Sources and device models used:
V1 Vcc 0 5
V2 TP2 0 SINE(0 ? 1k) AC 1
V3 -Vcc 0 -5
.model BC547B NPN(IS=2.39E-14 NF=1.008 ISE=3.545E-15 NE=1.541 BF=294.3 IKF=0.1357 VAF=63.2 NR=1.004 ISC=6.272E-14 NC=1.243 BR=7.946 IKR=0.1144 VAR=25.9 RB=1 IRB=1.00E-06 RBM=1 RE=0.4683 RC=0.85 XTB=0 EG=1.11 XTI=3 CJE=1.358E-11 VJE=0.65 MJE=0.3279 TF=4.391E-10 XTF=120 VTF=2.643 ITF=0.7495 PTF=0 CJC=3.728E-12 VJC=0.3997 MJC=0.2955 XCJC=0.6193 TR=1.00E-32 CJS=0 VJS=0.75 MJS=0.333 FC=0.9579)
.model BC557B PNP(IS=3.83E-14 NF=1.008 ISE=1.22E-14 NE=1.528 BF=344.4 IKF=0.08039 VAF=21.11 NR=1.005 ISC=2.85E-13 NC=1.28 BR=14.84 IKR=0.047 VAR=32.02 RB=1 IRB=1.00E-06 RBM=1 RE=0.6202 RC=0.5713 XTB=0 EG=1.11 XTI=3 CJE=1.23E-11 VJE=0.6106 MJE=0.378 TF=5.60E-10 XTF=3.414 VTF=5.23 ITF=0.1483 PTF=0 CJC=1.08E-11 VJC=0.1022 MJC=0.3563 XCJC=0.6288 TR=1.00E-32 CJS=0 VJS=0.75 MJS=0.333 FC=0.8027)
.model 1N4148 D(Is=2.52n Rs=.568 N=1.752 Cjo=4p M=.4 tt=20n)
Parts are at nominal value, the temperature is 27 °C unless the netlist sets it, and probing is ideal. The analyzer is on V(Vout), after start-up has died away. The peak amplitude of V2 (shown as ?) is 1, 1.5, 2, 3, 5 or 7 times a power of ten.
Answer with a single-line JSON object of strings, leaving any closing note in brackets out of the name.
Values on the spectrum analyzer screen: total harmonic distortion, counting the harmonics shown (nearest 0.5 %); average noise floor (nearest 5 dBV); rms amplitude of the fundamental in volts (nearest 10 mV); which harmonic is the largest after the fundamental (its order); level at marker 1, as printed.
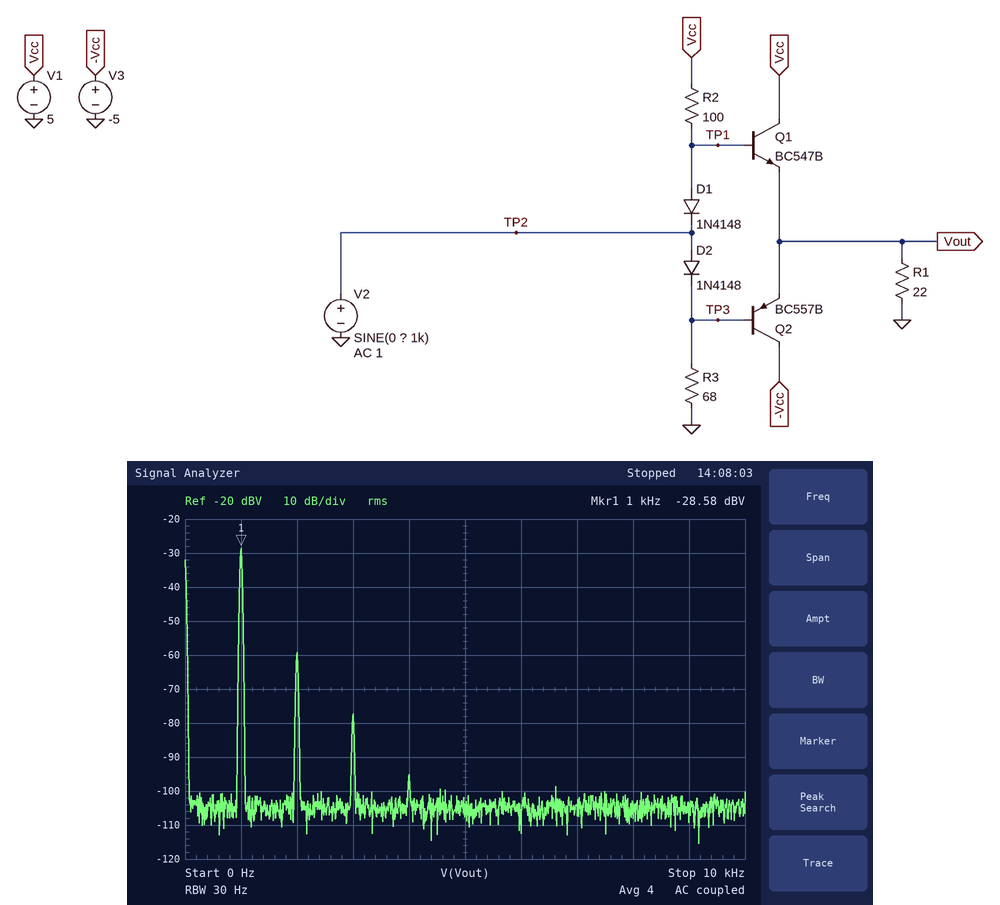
{"total harmonic distortion, counting the harmonics shown": "3.0 %", "average noise floor": "-105 dBV", "rms amplitude of the fundamental in volts": "40 mV", "which harmonic is the largest after the fundamental": "2", "level at marker 1, as printed": "-28.58 dBV"}
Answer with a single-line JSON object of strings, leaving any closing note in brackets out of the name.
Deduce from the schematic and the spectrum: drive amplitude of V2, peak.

{"drive amplitude of V2, peak": "70 mV"}
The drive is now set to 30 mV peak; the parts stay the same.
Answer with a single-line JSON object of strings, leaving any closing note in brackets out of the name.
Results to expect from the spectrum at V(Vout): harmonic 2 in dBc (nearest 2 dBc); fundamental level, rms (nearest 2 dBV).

{"harmonic 2 in dBc": "-38 dBc", "fundamental level, rms": "-36 dBV"}
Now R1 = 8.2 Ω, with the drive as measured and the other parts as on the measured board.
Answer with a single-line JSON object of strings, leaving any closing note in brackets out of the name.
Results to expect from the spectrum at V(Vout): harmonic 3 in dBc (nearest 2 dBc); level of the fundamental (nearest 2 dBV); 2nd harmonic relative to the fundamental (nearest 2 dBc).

{"harmonic 3 in dBc": "-46 dBc", "level of the fundamental": "-30 dBV", "2nd harmonic relative to the fundamental": "-28 dBc"}
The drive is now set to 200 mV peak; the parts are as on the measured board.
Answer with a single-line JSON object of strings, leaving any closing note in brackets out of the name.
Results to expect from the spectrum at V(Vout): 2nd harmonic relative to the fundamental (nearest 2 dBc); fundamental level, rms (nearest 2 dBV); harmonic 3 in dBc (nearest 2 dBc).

{"2nd harmonic relative to the fundamental": "-18 dBc", "fundamental level, rms": "-20 dBV", "harmonic 3 in dBc": "-28 dBc"}
